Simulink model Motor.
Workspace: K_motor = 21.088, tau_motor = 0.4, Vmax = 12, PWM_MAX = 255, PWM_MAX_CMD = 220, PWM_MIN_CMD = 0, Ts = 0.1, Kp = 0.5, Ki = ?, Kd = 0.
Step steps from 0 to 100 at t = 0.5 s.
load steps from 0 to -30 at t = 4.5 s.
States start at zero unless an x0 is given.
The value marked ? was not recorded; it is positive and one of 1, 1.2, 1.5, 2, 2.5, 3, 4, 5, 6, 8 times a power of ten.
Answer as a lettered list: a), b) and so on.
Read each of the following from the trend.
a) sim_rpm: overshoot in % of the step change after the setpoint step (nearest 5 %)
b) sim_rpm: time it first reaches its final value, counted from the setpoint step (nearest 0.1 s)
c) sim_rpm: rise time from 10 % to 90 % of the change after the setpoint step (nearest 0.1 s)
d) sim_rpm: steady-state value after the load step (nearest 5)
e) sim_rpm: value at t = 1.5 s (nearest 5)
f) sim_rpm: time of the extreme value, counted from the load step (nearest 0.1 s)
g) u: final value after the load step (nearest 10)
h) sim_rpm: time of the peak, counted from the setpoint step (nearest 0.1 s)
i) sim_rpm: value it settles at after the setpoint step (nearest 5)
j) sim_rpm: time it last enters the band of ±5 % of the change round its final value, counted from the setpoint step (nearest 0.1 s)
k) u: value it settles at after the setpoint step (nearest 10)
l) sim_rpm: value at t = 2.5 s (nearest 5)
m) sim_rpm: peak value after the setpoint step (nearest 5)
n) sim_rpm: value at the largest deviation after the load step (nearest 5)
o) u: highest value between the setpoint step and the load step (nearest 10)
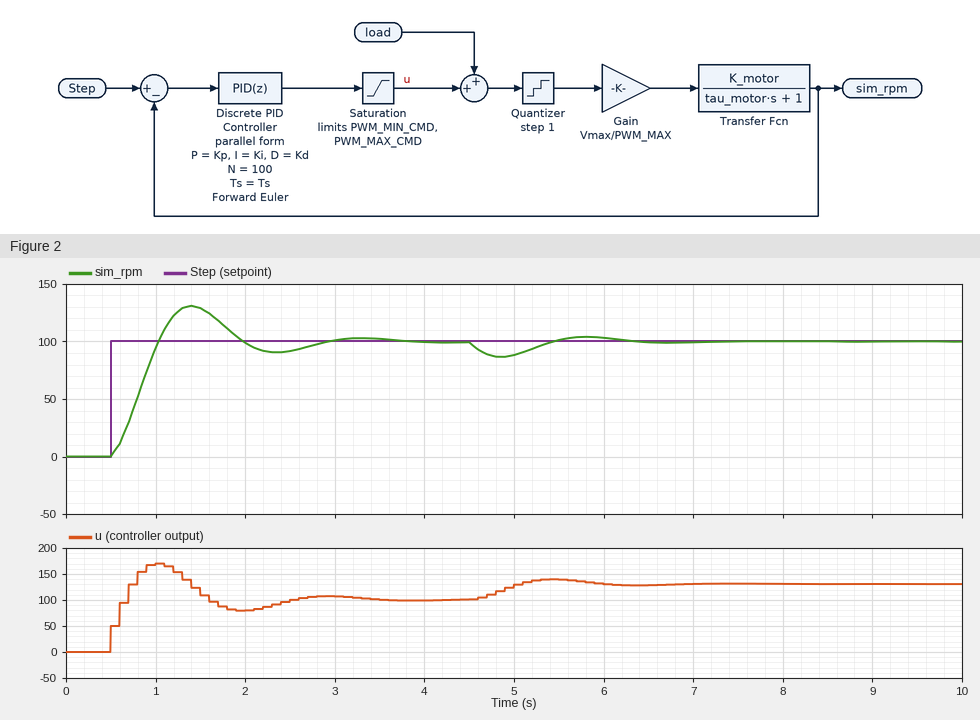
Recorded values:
a) 30 %
b) 0.5 s
c) 0.4 s
d) 100
e) 130
f) 0.4 s
g) 130
h) 0.9 s
i) 100
j) 2.2 s
k) 100
l) 90
m) 130
n) 85
o) 170
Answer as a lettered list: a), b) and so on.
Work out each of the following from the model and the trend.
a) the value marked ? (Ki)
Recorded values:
a) 5
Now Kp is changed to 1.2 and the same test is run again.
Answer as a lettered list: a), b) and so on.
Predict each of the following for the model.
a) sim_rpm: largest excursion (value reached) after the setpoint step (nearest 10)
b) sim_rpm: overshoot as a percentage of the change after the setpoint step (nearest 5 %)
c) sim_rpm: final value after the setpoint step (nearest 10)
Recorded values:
a) 110
b) 10 %
c) 100
